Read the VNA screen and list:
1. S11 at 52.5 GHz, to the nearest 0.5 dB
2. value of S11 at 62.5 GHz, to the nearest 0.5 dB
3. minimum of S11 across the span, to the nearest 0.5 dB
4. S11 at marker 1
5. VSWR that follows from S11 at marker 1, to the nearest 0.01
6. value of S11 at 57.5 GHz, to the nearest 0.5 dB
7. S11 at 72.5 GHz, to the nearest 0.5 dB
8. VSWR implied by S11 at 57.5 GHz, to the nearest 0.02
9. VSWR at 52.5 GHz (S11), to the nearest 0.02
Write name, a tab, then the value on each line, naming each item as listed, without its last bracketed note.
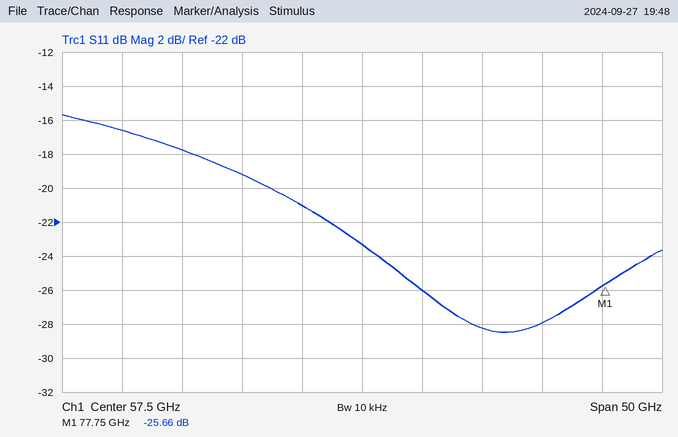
S11 at 52.5 GHz, to the nearest 0.5 dB	-21.0 dB
value of S11 at 62.5 GHz, to the nearest 0.5 dB	-26.0 dB
minimum of S11 across the span, to the nearest 0.5 dB	-28.5 dB
S11 at marker 1	-25.66 dB
VSWR that follows from S11 at marker 1, to the nearest 0.01	1.11
value of S11 at 57.5 GHz, to the nearest 0.5 dB	-23.5 dB
S11 at 72.5 GHz, to the nearest 0.5 dB	-28.0 dB
VSWR implied by S11 at 57.5 GHz, to the nearest 0.02	1.14
VSWR at 52.5 GHz (S11), to the nearest 0.02	1.20
